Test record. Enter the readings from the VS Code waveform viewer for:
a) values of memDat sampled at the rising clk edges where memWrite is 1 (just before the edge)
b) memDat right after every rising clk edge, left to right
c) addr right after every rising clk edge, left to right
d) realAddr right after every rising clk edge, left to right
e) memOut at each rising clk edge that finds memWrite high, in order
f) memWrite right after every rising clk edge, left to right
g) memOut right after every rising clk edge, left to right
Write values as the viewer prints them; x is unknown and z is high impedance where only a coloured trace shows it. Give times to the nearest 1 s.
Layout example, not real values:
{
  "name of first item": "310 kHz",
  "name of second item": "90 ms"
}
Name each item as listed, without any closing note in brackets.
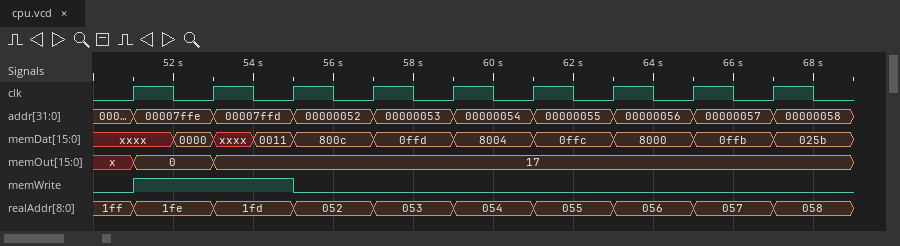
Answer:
{
  "values of memDat sampled at the rising clk edges where memWrite is 1": "0000, 0011",
  "memDat right after every rising clk edge, left to right": "xxxx, xxxx, 800c, 0ffd, 8004, 0ffc, 8000, 0ffb, 025b",
  "addr right after every rising clk edge, left to right": "00007ffe, 00007ffd, 00000052, 00000053, 00000054, 00000055, 00000056, 00000057, 00000058",
  "realAddr right after every rising clk edge, left to right": "1fe, 1fd, 052, 053, 054, 055, 056, 057, 058",
  "memOut at each rising clk edge that finds memWrite high, in order": "0, 17",
  "memWrite right after every rising clk edge, left to right": "1 1 0 0 0 0 0 0 0",
  "memOut right after every rising clk edge, left to right": "0, 17, 17, 17, 17, 17, 17, 17, 17"
}
